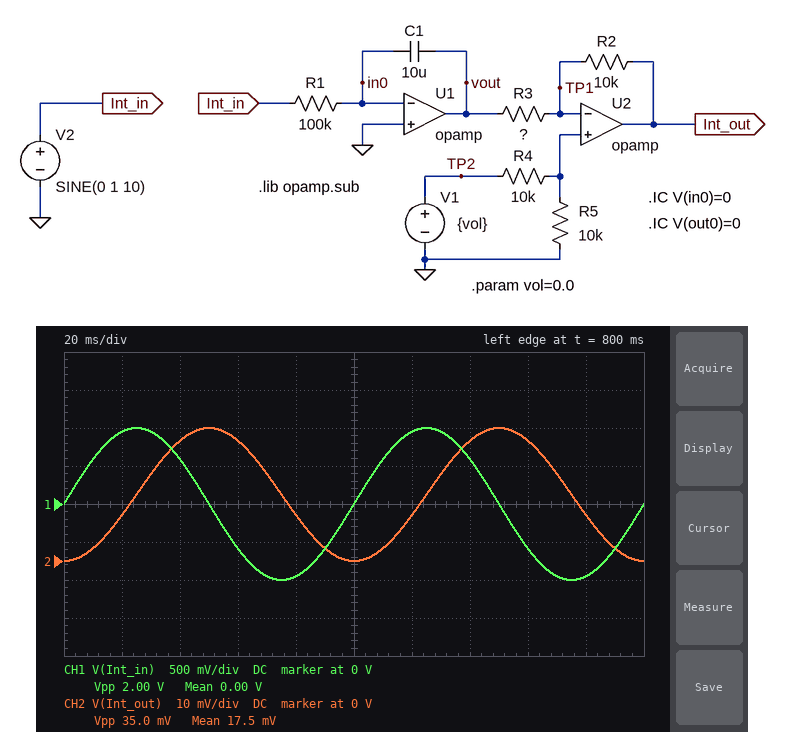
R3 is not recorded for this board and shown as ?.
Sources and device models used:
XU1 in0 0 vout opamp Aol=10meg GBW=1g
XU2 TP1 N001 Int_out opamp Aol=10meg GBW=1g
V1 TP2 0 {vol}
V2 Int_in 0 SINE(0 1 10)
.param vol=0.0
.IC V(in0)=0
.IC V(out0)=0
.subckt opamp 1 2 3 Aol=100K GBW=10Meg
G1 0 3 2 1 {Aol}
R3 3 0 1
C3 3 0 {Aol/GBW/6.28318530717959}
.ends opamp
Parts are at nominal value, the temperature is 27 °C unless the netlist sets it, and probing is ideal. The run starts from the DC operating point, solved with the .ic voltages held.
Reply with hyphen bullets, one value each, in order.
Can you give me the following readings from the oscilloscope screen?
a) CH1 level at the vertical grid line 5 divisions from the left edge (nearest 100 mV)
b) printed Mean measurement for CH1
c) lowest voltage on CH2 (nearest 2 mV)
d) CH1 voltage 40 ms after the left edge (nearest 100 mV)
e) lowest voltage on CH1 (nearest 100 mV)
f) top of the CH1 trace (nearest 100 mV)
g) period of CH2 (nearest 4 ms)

- 0 V
- 0.00 V
- 0 V
- 600 mV
- -1.0 V
- 1.0 V
- 100 ms
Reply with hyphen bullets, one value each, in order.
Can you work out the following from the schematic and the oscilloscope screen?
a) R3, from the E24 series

- 9.1 kΩ
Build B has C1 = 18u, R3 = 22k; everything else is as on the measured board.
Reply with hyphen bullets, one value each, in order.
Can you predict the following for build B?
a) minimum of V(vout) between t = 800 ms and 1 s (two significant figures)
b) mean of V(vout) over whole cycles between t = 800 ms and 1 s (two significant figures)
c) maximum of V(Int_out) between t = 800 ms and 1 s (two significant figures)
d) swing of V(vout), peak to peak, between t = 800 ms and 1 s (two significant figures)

- -18 mV
- -8.8 mV
- 8.0 mV
- 18 mV
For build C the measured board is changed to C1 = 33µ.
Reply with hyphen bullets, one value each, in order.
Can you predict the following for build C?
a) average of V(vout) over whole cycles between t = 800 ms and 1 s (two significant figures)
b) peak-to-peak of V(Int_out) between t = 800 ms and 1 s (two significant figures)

- -4.8 mV
- 11 mV
